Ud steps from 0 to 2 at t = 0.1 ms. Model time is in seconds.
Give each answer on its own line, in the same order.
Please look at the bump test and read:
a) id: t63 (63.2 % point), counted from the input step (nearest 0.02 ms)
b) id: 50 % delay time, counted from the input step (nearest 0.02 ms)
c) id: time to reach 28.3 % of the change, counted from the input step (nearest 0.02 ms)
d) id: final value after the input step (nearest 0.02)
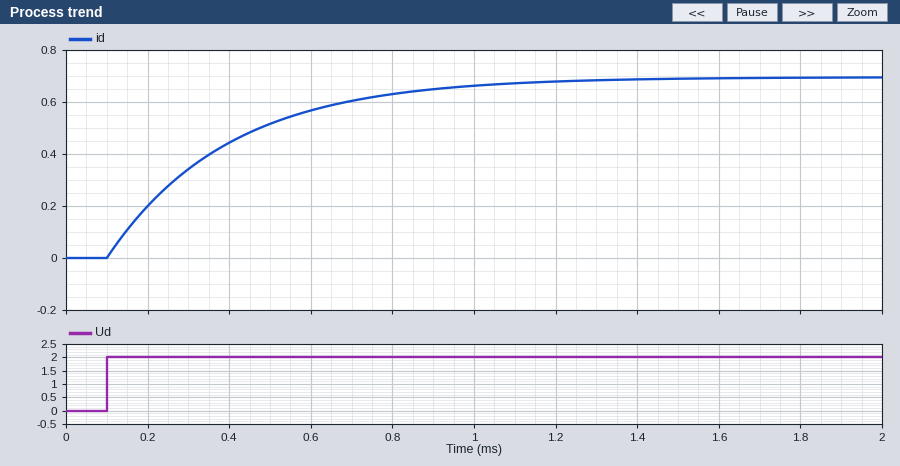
0.30 ms
0.20 ms
0.10 ms
0.70
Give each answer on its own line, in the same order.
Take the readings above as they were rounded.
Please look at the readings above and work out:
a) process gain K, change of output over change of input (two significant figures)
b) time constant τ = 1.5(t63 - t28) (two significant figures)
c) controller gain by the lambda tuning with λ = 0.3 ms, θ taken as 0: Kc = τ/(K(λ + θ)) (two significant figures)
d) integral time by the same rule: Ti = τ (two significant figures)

0.35
0.30 ms
2.9
0.30 ms
